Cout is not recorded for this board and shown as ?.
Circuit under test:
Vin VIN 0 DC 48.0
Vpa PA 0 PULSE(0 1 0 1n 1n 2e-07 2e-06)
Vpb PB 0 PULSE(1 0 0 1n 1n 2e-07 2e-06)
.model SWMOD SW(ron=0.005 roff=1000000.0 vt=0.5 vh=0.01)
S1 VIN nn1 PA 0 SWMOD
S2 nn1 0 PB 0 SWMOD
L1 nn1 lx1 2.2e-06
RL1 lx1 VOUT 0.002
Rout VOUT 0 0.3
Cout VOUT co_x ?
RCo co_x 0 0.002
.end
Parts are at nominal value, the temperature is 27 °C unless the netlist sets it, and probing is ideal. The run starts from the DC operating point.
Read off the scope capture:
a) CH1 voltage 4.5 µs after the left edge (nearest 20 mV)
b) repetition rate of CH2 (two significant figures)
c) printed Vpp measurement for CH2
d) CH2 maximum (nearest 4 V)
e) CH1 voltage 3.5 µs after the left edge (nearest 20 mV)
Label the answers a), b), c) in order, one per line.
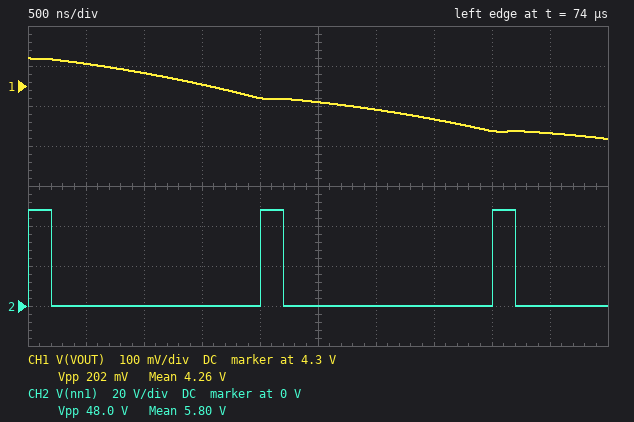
a) 4.18 V
b) 500 kHz
c) 48.0 V
d) 48 V
e) 4.22 V
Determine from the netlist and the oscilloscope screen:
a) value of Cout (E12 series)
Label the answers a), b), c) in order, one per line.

a) 82 µF
